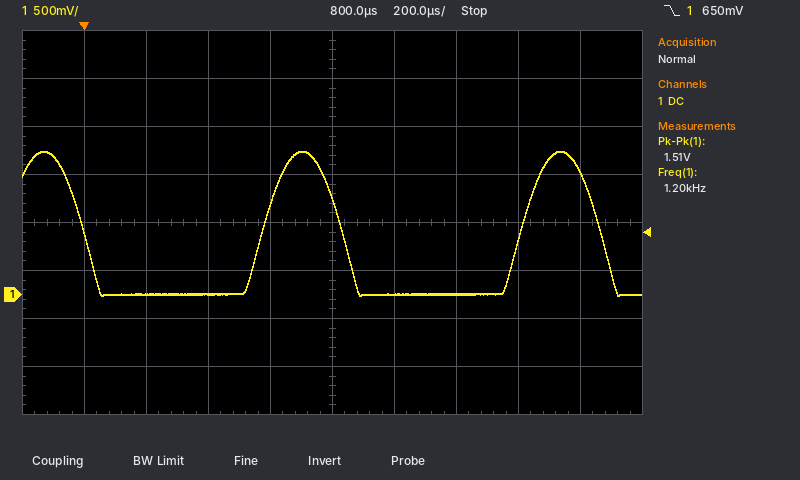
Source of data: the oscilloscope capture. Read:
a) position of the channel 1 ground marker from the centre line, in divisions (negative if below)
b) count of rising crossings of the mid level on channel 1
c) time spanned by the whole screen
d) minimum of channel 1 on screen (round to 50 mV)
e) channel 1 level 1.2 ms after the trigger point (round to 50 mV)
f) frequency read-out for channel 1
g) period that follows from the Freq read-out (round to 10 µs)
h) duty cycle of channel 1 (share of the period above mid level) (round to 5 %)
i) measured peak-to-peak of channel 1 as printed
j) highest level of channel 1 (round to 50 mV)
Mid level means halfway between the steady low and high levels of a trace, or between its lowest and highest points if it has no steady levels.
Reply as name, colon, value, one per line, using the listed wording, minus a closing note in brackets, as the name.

position of the channel 1 ground marker from the centre line, in divisions: -1.5 div
count of rising crossings of the mid level on channel 1: 2
time spanned by the whole screen: 2 ms
minimum of channel 1 on screen: 0 mV
channel 1 level 1.2 ms after the trigger point: 0 mV
frequency read-out for channel 1: 1.20 kHz
period that follows from the Freq read-out: 830 µs
duty cycle of channel 1 (share of the period above mid level): 30 %
measured peak-to-peak of channel 1 as printed: 1.51 V
highest level of channel 1: 1.50 V
